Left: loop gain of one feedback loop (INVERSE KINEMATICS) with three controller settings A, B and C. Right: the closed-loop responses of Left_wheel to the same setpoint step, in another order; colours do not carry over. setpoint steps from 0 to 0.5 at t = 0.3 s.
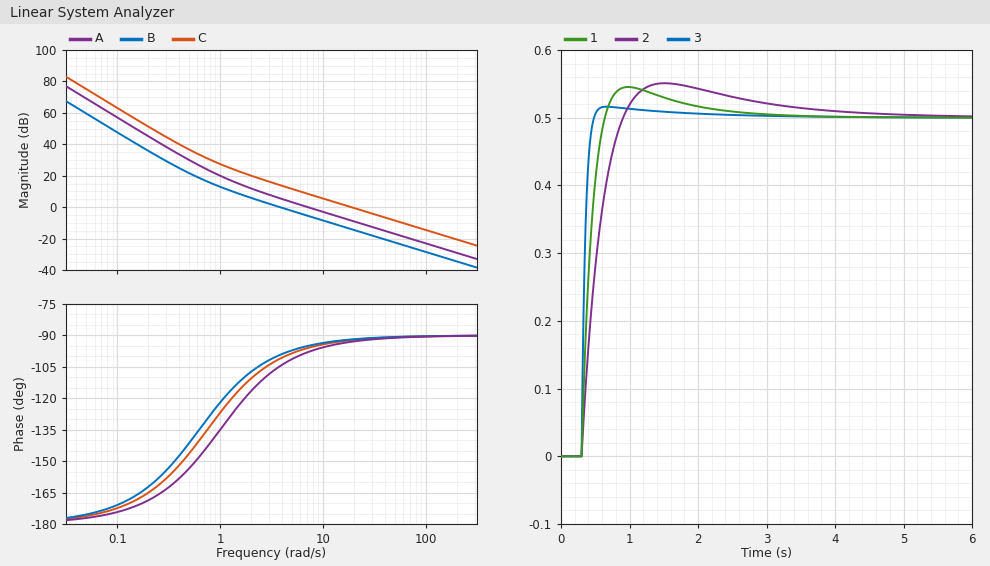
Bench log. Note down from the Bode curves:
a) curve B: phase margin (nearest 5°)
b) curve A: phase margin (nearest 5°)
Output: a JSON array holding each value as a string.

["80°", "80°"]
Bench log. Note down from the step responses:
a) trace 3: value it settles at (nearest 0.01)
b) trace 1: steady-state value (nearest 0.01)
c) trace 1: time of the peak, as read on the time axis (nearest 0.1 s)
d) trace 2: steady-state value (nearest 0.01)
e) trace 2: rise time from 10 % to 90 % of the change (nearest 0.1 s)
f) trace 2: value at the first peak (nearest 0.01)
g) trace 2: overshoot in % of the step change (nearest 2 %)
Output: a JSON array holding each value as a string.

["0.50", "0.50", "1.0 s", "0.50", "0.4 s", "0.55", "10 %"]
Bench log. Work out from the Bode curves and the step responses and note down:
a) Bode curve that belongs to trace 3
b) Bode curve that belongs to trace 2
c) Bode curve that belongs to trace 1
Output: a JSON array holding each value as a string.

["C", "B", "A"]
